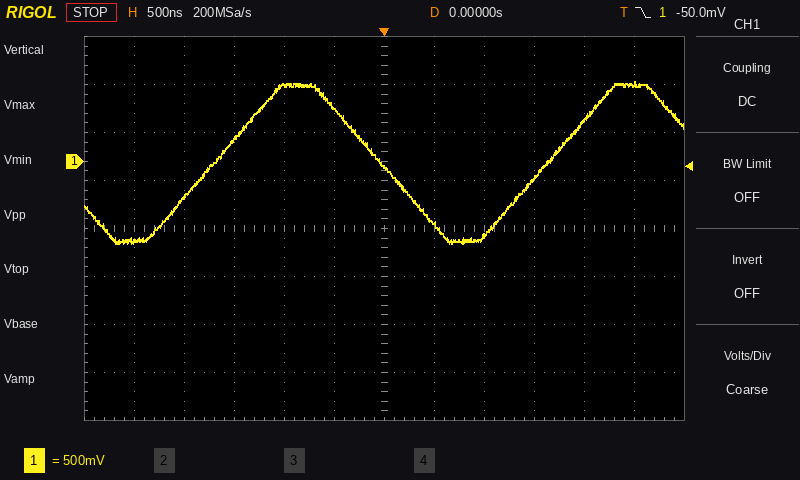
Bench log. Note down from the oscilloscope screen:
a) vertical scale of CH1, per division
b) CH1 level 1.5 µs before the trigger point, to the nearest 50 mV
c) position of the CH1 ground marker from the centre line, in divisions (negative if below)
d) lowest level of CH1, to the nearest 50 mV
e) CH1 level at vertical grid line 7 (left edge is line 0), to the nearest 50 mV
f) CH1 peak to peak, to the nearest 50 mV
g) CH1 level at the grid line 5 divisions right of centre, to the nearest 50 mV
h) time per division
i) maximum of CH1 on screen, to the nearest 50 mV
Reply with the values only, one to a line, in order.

500 mV
250 mV
+1.4 div
-850 mV
-650 mV
1.70 V
800 mV
500 ns
850 mV
